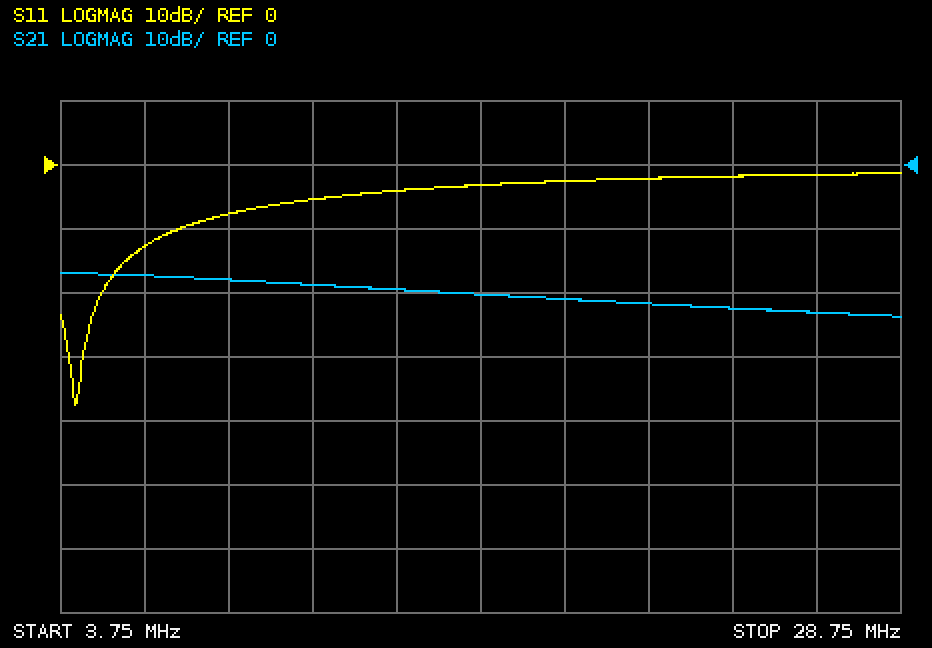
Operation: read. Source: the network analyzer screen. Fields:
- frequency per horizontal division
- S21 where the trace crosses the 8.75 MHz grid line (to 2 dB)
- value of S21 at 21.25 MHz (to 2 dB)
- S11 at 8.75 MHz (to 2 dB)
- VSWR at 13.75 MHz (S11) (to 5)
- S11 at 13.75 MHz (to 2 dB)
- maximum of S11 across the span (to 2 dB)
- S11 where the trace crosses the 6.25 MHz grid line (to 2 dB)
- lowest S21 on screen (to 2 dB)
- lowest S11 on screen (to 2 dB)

2.5 MHz
-18 dB
-22 dB
-8 dB
5
-4 dB
-2 dB
-12 dB
-24 dB
-38 dB
